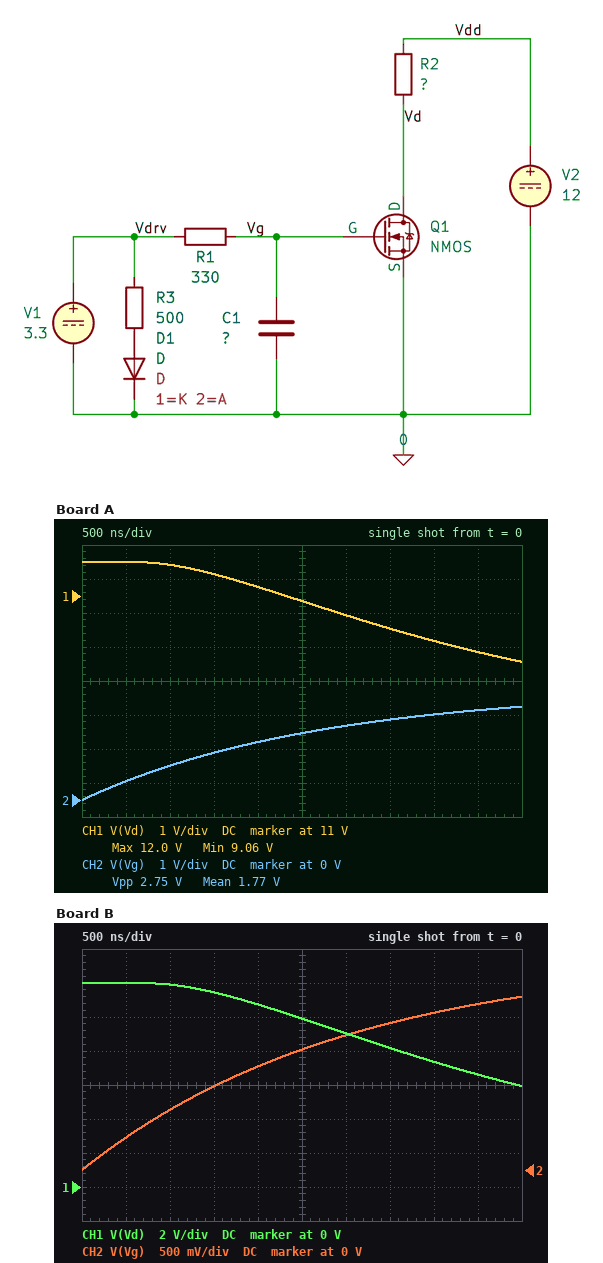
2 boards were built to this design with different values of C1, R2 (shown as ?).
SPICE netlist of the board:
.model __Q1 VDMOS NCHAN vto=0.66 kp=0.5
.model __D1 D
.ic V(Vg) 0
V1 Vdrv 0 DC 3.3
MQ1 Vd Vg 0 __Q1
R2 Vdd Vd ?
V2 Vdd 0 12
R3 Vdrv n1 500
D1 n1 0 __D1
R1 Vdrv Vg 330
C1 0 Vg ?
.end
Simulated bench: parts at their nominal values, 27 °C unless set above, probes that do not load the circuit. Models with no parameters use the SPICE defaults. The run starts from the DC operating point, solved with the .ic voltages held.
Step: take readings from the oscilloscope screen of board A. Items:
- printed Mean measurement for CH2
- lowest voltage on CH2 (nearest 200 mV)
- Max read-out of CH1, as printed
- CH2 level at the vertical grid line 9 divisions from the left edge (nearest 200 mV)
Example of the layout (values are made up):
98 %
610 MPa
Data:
1.77 V
0 V
12.0 V
2.6 V
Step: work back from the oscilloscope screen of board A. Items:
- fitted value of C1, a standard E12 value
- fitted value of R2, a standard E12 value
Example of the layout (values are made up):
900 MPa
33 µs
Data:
6.8 nF
2.7 Ω
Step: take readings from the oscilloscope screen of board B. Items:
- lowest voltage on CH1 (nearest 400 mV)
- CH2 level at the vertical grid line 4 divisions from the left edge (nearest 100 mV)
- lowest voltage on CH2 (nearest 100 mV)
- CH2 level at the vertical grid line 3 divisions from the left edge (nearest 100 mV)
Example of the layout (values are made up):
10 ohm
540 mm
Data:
6.0 V
1.5 V
0 V
1.2 V
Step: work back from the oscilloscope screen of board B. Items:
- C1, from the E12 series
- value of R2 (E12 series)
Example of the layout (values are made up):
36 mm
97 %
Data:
8.2 nF
6.8 Ω
